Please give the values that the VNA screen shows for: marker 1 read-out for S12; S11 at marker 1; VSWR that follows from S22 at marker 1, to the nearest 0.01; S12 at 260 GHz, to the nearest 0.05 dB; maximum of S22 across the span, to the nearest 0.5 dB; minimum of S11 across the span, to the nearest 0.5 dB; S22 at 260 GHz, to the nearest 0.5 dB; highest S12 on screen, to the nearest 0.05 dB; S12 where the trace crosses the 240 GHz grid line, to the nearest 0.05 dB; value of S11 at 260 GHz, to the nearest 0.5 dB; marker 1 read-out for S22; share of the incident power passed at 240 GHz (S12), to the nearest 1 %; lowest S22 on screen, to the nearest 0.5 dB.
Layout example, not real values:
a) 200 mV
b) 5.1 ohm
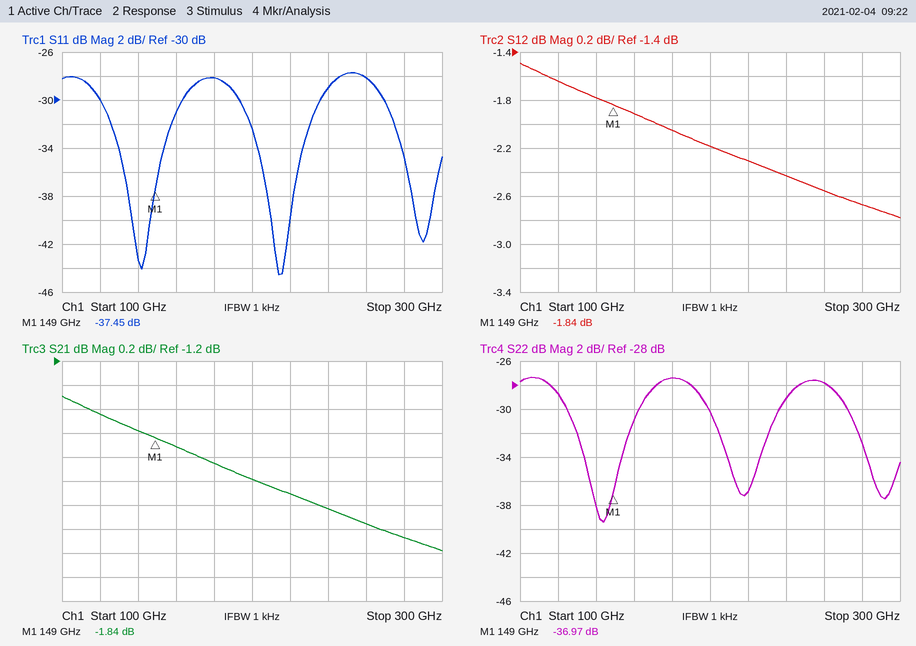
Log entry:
a) -1.84 dB
b) -37.45 dB
c) 1.03
d) -2.55 dB
e) -27.5 dB
f) -44.5 dB
g) -28.0 dB
h) -1.50 dB
i) -2.45 dB
j) -28.0 dB
k) -36.97 dB
l) 57 %
m) -39.5 dB
